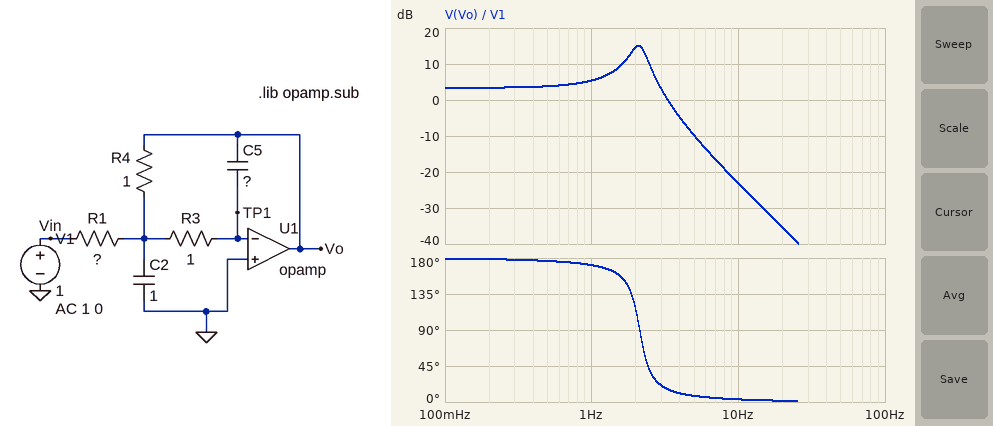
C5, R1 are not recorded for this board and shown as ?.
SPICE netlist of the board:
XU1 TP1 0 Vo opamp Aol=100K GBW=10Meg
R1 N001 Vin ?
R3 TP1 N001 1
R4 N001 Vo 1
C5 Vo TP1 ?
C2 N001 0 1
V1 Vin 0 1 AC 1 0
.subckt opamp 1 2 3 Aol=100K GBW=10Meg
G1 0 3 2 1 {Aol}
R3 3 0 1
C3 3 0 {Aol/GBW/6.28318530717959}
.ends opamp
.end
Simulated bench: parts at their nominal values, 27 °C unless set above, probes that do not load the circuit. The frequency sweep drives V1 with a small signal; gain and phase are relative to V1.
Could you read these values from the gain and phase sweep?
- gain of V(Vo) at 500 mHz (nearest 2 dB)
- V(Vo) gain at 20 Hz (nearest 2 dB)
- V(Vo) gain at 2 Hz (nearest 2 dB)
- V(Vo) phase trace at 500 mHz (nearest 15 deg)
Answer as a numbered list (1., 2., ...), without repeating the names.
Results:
1. 4 dB
2. -36 dB
3. 14 dB
4. 180 deg
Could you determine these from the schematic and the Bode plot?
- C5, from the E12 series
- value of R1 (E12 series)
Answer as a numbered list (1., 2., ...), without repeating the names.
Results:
1. 5.6 mF
2. 0.68 Ω
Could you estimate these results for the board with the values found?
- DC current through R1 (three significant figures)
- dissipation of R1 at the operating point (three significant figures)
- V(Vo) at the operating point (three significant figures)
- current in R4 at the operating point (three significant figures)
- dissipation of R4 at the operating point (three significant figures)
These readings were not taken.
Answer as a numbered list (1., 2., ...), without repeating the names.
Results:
1. 1.47 A
2. 1.47 W
3. -1.47 V
4. 1.47 A
5. 2.16 W
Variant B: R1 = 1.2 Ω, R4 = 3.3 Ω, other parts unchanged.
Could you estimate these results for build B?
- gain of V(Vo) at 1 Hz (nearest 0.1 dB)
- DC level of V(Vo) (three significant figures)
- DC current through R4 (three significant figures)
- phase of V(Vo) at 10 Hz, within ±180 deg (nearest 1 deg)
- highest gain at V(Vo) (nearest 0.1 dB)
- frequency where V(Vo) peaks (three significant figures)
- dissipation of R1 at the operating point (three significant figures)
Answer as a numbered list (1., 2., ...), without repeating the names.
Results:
1. 17.5 dB
2. -2.75 V
3. 833 mA
4. 2 deg
5. 19.6 dB
6. 1.15 Hz
7. 833 mW
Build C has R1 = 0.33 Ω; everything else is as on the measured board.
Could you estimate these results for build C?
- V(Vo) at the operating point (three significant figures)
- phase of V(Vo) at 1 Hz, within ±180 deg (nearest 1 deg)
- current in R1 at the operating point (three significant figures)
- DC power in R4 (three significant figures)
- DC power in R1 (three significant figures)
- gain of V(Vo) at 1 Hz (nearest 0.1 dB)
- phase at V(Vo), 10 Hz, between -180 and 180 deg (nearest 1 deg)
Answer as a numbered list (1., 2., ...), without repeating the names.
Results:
1. -3.03 V
2. 167 deg
3. 3.03 A
4. 9.18 W
5. 3.03 W
6. 11.6 dB
7. 5 deg
